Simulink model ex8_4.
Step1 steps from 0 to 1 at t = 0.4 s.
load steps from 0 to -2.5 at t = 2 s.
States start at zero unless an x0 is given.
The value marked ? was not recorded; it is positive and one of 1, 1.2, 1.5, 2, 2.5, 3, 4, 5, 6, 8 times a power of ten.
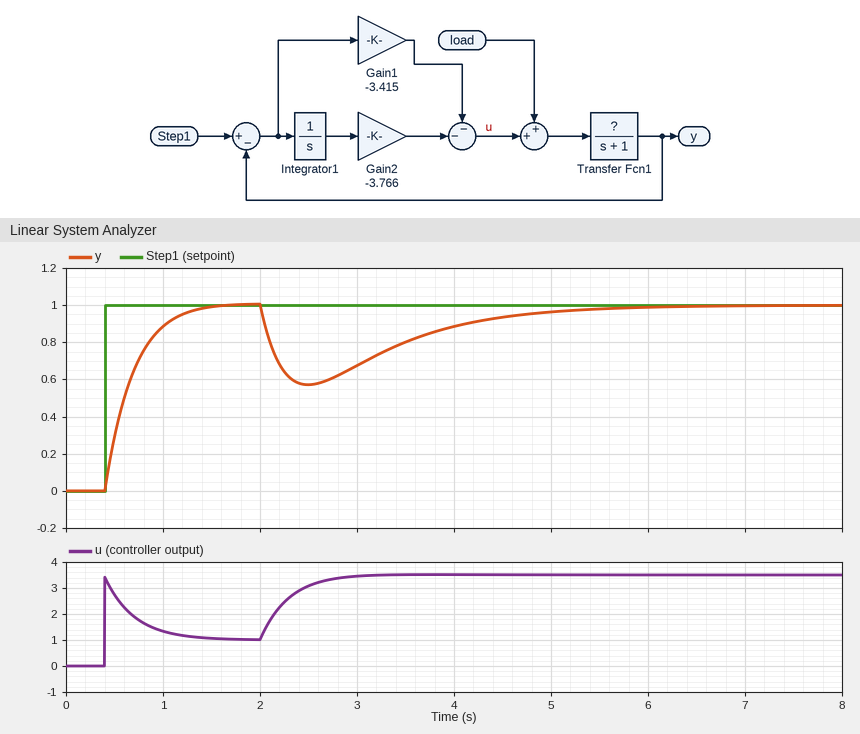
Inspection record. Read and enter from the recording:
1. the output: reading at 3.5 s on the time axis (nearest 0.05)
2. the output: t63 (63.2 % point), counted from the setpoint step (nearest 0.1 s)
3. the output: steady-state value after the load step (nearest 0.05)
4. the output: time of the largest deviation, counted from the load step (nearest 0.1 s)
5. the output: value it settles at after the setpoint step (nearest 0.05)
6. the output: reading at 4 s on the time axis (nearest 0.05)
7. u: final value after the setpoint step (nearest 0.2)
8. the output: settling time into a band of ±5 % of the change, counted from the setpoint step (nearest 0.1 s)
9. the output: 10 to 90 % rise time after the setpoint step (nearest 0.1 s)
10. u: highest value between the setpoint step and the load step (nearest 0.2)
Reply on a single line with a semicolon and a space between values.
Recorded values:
0.80; 0.3 s; 1.00; 0.5 s; 1.00; 0.90; 1.0; 0.8 s; 0.6 s; 3.4
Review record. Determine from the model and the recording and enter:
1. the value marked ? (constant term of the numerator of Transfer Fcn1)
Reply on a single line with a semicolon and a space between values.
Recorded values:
1
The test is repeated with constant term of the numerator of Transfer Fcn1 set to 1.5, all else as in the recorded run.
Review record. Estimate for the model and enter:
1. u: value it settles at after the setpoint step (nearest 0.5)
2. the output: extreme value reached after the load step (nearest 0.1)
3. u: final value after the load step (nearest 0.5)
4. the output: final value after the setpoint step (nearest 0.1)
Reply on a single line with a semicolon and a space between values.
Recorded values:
0.5; 0.5; 3.0; 1.0
